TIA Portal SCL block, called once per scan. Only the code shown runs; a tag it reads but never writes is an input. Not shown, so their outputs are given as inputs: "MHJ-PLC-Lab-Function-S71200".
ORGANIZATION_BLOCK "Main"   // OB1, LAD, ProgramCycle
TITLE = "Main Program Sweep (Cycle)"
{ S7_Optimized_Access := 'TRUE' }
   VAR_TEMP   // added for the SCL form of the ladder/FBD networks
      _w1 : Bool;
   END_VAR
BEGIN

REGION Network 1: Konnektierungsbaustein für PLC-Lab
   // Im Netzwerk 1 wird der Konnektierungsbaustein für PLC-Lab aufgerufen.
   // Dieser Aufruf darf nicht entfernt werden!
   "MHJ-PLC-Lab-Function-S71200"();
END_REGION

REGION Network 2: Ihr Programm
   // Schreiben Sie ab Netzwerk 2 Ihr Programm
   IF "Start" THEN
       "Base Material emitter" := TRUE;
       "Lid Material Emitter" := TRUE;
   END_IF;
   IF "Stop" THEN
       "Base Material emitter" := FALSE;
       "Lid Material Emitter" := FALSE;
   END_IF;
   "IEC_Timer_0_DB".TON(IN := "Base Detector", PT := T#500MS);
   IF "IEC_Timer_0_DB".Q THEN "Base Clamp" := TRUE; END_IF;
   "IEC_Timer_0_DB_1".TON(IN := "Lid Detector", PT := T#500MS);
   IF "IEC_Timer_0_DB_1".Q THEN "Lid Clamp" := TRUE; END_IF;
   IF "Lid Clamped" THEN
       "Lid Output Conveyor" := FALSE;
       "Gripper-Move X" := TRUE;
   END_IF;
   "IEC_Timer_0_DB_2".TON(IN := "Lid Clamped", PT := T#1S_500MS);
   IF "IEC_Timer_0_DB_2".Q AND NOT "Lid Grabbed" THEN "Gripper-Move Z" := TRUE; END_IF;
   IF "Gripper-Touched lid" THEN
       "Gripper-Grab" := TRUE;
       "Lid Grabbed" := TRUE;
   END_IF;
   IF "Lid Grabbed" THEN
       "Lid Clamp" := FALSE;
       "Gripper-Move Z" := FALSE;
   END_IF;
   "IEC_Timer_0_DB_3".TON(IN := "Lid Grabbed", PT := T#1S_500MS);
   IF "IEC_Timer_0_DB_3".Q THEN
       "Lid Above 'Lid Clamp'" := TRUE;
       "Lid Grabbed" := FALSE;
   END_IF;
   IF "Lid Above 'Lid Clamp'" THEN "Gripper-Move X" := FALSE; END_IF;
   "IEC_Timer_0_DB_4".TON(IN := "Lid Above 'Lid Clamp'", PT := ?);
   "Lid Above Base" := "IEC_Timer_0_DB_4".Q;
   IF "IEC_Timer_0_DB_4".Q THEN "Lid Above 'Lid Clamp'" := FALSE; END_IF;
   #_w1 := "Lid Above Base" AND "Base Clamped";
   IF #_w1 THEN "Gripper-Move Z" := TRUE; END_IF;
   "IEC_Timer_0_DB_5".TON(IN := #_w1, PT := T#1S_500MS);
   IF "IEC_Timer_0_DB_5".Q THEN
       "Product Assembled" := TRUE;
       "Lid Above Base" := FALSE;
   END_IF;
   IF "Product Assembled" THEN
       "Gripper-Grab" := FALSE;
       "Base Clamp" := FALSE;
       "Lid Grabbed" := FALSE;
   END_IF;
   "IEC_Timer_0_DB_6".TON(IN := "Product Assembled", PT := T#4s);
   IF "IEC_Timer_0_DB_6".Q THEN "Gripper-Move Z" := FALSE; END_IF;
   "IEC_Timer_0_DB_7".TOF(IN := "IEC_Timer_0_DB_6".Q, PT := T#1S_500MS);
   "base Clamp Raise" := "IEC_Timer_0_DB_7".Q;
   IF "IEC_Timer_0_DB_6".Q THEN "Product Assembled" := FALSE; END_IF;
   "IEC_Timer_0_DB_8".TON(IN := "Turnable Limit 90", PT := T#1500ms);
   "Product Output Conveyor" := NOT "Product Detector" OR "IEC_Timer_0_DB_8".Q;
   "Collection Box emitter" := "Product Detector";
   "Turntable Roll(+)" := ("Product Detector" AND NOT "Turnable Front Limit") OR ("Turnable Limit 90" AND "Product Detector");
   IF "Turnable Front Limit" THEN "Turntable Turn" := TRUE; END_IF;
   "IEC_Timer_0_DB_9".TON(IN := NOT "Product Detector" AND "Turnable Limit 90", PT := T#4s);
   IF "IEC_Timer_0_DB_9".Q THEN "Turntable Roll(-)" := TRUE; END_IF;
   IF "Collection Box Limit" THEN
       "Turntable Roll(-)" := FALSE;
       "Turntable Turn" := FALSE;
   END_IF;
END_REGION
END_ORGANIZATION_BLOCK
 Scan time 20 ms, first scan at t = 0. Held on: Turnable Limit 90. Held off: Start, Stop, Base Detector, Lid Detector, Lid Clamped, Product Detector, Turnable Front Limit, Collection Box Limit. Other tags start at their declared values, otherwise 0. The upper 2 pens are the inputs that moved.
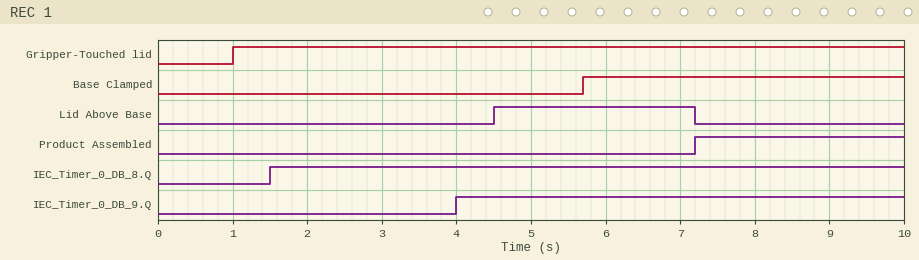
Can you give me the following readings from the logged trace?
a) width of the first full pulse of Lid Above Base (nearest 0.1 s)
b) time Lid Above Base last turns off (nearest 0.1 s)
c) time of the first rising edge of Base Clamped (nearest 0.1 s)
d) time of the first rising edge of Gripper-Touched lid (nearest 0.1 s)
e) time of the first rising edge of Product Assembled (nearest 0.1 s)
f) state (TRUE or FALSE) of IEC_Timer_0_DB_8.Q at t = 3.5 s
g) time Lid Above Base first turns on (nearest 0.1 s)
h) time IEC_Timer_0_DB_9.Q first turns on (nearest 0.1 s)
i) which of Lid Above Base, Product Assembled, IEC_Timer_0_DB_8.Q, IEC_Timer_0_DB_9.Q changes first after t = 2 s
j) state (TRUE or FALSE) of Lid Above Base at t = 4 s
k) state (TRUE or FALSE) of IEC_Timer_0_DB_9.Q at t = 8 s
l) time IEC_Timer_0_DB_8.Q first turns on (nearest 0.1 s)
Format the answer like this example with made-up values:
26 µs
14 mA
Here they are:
2.7 s
7.2 s
5.7 s
1.0 s
7.2 s
TRUE
4.5 s
4.0 s
IEC_Timer_0_DB_9.Q
FALSE
TRUE
1.5 s
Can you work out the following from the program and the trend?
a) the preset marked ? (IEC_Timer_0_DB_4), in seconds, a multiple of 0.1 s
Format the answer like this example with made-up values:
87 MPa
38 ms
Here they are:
2.0 s
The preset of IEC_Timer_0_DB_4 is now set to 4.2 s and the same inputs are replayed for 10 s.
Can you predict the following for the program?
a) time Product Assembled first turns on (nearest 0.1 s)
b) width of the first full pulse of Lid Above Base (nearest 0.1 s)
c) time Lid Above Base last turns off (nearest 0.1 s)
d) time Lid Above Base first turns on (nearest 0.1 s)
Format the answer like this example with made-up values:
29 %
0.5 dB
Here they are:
8.2 s
1.5 s
8.2 s
6.7 s
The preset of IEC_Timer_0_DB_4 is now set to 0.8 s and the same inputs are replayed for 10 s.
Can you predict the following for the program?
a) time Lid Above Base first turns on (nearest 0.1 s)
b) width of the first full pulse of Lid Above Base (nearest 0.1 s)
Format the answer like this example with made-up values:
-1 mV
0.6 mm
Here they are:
3.3 s
3.9 s
